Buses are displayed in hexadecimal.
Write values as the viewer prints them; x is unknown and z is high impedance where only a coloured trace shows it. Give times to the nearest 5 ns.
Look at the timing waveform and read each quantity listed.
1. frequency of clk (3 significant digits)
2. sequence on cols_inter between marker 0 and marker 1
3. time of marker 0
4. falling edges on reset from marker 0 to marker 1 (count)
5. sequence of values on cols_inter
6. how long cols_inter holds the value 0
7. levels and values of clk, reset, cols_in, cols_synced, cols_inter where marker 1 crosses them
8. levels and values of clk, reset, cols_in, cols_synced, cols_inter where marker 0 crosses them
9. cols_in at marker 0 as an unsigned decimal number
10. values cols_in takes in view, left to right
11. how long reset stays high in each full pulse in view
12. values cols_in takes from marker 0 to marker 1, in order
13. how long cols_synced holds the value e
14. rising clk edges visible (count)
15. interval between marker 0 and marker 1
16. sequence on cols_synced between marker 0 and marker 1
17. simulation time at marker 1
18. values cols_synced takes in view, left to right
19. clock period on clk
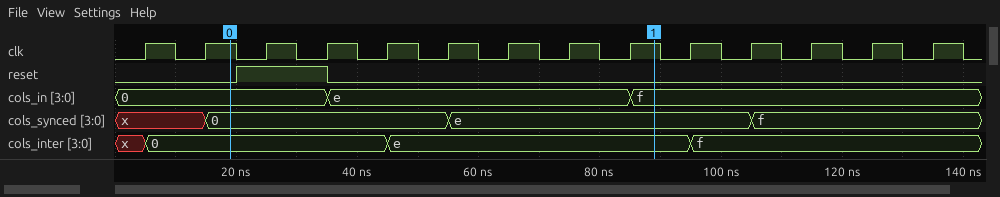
100 MHz
0, e
20 ns
1
x, 0, e, f
40 ns
clk=1, reset=0, cols_in=f, cols_synced=e, cols_inter=e
clk=1, reset=0, cols_in=0, cols_synced=0, cols_inter=0
0
0, e, f
15 ns
0, e, f
50 ns
14
70 ns
0, e
90 ns
x, 0, e, f
10 ns
